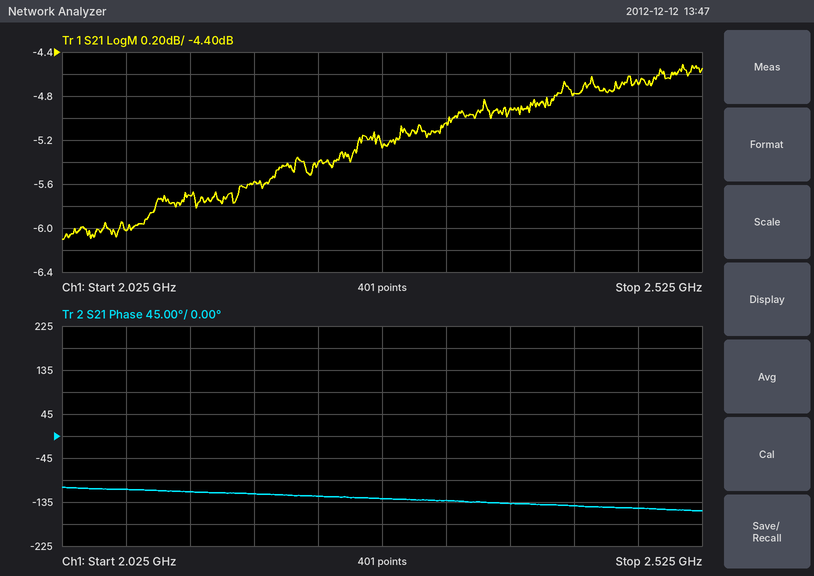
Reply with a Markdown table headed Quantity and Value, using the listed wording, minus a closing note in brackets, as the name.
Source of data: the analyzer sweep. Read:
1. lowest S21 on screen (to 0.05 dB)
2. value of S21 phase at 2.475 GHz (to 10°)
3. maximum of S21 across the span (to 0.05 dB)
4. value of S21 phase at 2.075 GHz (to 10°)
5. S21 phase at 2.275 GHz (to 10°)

| Quantity | Value |
|---|---|
| lowest S21 on screen | -6.10 dB |
| value of S21 phase at 2.475 GHz | -150° |
| maximum of S21 across the span | -4.50 dB |
| value of S21 phase at 2.075 GHz | -110° |
| S21 phase at 2.275 GHz | -130° |
